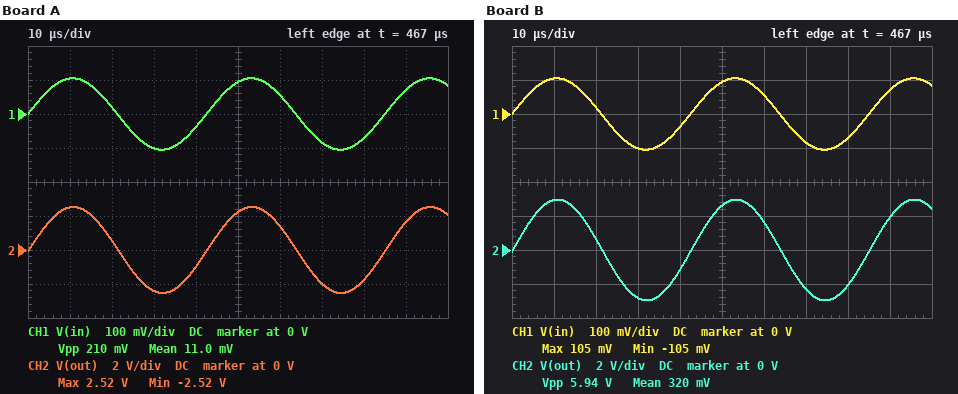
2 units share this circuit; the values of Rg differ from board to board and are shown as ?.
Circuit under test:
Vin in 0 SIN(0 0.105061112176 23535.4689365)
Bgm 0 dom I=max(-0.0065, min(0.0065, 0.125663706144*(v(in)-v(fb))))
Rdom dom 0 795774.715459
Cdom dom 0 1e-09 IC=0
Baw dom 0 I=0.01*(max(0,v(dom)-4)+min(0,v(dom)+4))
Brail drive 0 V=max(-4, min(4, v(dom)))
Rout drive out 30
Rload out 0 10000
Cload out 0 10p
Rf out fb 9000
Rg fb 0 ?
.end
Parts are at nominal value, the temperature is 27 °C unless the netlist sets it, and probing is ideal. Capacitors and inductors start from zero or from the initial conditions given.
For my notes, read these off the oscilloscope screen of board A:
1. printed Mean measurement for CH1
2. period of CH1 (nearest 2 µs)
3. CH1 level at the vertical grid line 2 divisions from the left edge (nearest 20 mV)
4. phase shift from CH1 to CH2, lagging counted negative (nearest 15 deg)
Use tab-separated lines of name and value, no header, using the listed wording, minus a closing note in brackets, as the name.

printed Mean measurement for CH1	11.0 mV
period of CH1	42 µs
CH1 level at the vertical grid line 2 divisions from the left edge	20 mV
phase shift from CH1 to CH2, lagging counted negative	0 deg
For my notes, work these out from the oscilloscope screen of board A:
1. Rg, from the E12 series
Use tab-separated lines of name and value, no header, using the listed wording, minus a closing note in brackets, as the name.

Rg, from the E12 series	390 Ω
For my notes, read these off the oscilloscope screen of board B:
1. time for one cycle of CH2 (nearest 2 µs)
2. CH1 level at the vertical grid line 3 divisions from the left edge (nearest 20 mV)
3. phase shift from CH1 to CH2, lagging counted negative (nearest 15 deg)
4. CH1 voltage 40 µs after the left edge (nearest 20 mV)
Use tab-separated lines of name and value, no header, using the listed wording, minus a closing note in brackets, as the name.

time for one cycle of CH2	42 µs
CH1 level at the vertical grid line 3 divisions from the left edge	-100 mV
phase shift from CH1 to CH2, lagging counted negative	0 deg
CH1 voltage 40 µs after the left edge	-40 mV
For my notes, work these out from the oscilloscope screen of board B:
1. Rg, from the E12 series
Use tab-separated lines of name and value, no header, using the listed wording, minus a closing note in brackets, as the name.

Rg, from the E12 series	330 Ω
